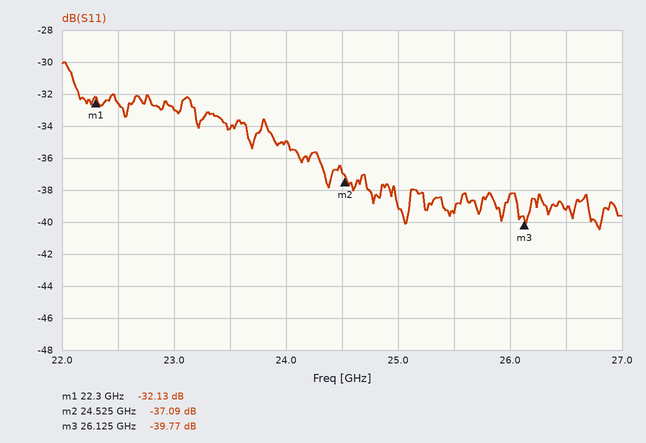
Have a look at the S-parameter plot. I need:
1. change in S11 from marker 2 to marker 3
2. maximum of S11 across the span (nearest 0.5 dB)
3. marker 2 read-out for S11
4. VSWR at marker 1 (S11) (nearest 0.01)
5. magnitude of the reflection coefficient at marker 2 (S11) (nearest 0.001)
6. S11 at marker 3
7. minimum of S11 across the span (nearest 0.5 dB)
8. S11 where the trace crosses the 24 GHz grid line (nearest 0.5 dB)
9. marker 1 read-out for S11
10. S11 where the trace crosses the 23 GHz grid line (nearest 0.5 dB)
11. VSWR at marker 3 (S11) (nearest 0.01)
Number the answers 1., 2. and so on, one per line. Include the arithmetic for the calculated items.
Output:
1. -39.77 − (-37.09) = -2.68 dB
2. -30.0 dB
3. -37.09 dB
4. (1 + 0.0247)/(1 − 0.0247) ≈ 1.05
5. 10^(-37.09/20) ≈ 0.014
6. -39.77 dB
7. -40.5 dB
8. -35.0 dB
9. -32.13 dB
10. -33.0 dB
11. (1 + 0.0103)/(1 − 0.0103) ≈ 1.02
